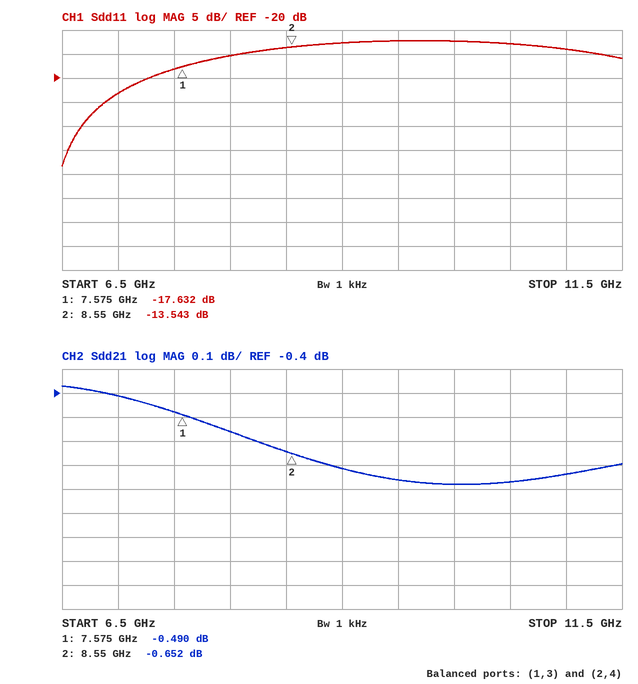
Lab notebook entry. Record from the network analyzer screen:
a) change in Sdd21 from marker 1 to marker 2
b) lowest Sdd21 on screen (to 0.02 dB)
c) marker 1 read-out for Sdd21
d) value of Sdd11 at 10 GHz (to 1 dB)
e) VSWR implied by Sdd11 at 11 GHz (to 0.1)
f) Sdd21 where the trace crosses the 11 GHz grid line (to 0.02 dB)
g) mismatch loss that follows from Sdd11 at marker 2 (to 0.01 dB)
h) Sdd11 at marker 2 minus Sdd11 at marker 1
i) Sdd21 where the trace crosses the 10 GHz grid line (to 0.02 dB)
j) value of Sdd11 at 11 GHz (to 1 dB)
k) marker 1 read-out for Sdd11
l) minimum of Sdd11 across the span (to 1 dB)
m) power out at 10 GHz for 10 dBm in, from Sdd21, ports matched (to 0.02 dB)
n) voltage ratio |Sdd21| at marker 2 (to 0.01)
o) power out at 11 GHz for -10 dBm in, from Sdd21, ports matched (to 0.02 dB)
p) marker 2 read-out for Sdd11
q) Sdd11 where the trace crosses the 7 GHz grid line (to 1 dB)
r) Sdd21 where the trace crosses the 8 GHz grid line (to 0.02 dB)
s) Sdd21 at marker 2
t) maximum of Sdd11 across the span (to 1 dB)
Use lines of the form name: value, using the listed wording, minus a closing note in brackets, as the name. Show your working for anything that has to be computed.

change in Sdd21 from marker 1 to marker 2: -0.652 − (-0.49) = -0.162 dB
lowest Sdd21 on screen: -0.78 dB
marker 1 read-out for Sdd21: -0.490 dB
value of Sdd11 at 10 GHz: -12 dB
VSWR implied by Sdd11 at 11 GHz: |Γ| = 10^(-14/20) = 0.1995; VSWR = (1 + 0.1995)/(1 − 0.1995) ≈ 1.5
Sdd21 where the trace crosses the 11 GHz grid line: -0.74 dB
mismatch loss that follows from Sdd11 at marker 2: −10 log10(1 − 10^(-13.543/10)) ≈ 0.20 dB
Sdd11 at marker 2 minus Sdd11 at marker 1: -13.543 − (-17.632) = 4.089 dB
Sdd21 where the trace crosses the 10 GHz grid line: -0.78 dB
value of Sdd11 at 11 GHz: -14 dB
marker 1 read-out for Sdd11: -17.632 dB
minimum of Sdd11 across the span: -38 dB
power out at 10 GHz for 10 dBm in, from Sdd21, ports matched: 10 dBm + (-0.78 dB) = 9.22 dBm
voltage ratio |Sdd21| at marker 2: 10^(-0.652/20) ≈ 0.93
power out at 11 GHz for -10 dBm in, from Sdd21, ports matched: -10 dBm + (-0.74 dB) = -10.74 dBm
marker 2 read-out for Sdd11: -13.543 dB
Sdd11 where the trace crosses the 7 GHz grid line: -23 dB
Sdd21 where the trace crosses the 8 GHz grid line: -0.56 dB
Sdd21 at marker 2: -0.652 dB
maximum of Sdd11 across the span: -12 dB
